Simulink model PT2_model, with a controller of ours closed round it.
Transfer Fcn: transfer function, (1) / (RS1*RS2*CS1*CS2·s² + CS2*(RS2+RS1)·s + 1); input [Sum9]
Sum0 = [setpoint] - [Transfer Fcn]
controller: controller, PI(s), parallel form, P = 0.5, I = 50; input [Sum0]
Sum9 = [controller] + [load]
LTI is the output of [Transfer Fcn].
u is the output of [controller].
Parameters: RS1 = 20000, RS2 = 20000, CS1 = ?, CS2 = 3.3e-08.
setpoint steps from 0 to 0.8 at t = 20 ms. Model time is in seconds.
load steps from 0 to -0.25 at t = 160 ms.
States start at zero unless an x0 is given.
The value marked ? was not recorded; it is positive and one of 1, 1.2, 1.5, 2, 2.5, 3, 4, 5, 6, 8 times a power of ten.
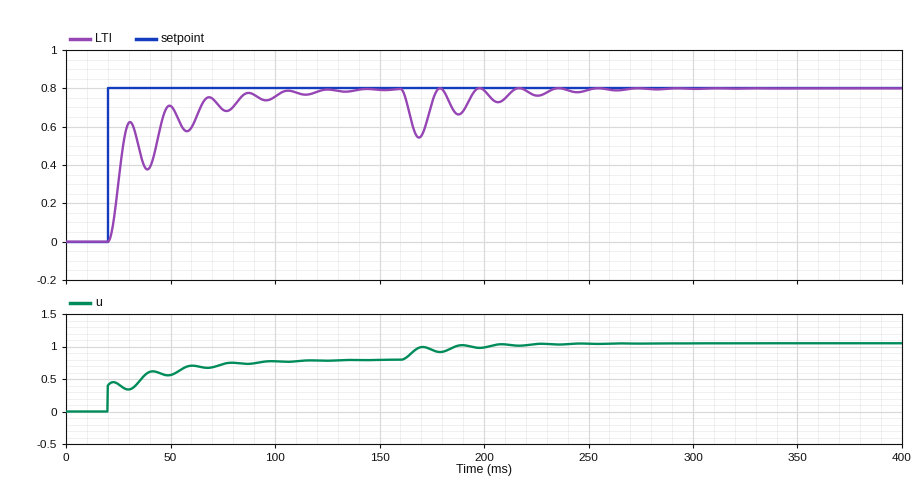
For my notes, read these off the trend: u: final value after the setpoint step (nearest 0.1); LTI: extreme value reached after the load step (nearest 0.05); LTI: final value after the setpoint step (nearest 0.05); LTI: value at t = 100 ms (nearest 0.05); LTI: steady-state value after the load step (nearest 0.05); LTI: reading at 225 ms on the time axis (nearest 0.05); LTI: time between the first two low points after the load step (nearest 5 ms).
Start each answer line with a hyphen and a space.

- 0.8
- 0.55
- 0.80
- 0.75
- 0.80
- 0.75
- 20 ms
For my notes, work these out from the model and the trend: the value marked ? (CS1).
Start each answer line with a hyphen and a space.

- 1e-06
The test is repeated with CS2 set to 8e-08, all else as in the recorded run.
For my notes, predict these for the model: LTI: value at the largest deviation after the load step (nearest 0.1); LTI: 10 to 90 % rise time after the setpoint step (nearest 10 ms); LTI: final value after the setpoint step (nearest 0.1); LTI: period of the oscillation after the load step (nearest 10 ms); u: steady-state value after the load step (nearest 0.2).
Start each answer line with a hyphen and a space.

- 0.6
- 40 ms
- 0.8
- 30 ms
- 1.0
